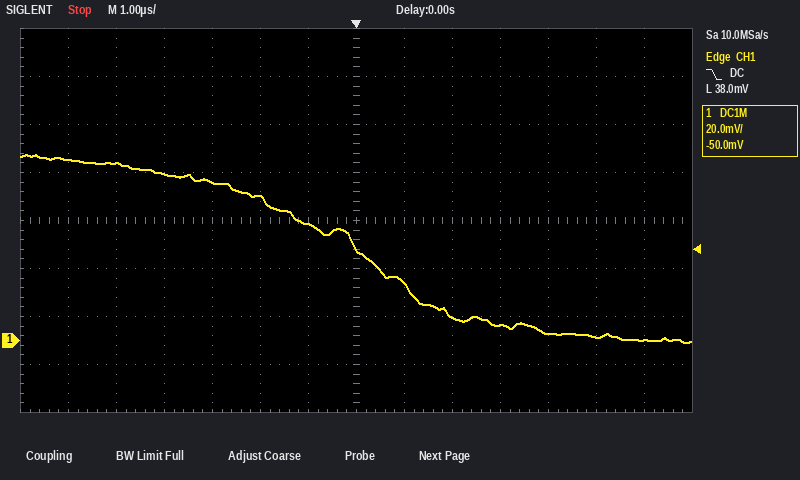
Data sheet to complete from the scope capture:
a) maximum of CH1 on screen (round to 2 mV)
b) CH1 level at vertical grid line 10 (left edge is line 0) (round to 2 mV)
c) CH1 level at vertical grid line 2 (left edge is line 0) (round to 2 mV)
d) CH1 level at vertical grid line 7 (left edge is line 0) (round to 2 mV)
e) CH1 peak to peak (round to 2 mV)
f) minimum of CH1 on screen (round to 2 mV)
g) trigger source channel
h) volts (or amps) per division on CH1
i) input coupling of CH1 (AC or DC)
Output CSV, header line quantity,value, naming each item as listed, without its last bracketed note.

quantity,value
maximum of CH1 on screen,78 mV
CH1 level at vertical grid line 10 (left edge is line 0),6 mV
CH1 level at vertical grid line 2 (left edge is line 0),74 mV
CH1 level at vertical grid line 7 (left edge is line 0),38 mV
CH1 peak to peak,78 mV
minimum of CH1 on screen,0 mV
trigger source channel,CH1
volts (or amps) per division on CH1,20 mV
input coupling of CH1,DC
